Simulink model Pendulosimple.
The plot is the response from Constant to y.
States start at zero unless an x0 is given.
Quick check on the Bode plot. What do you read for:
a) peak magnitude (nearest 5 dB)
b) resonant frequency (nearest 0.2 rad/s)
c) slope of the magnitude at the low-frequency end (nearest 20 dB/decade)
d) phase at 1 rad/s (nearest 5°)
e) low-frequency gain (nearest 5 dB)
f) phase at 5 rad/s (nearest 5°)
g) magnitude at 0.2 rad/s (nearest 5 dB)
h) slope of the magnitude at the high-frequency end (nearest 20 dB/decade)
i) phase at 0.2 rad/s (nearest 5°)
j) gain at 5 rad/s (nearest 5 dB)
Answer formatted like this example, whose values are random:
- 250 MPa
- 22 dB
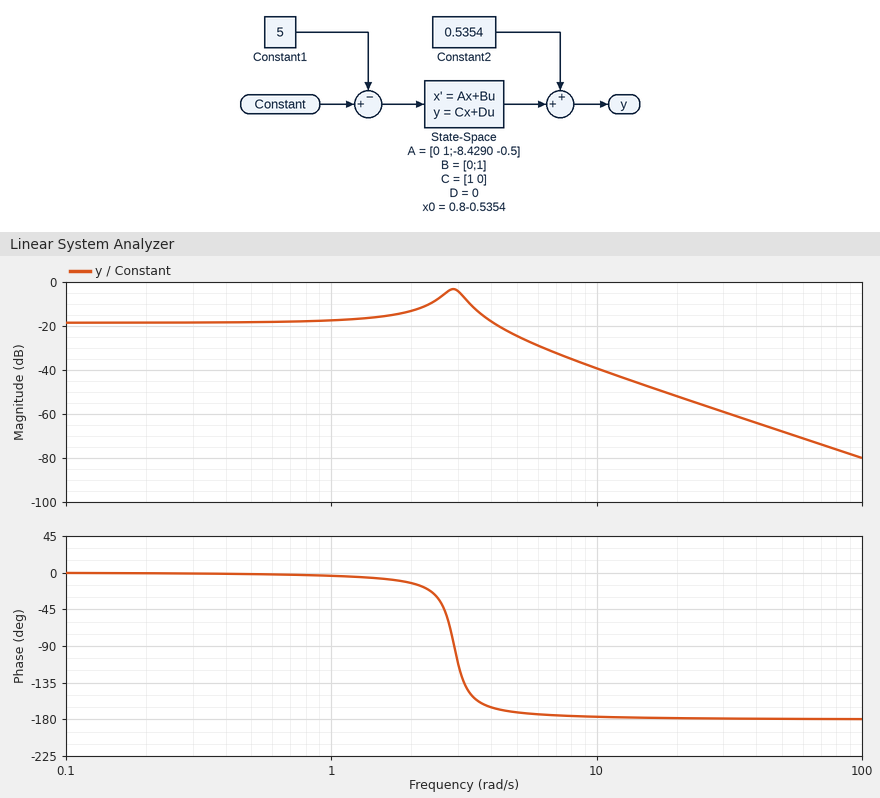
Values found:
- -5 dB
- 2.8 rad/s
- 0 dB/decade
- -5°
- -20 dB
- -170°
- -20 dB
- -40 dB/decade
- 0°
- -25 dB
